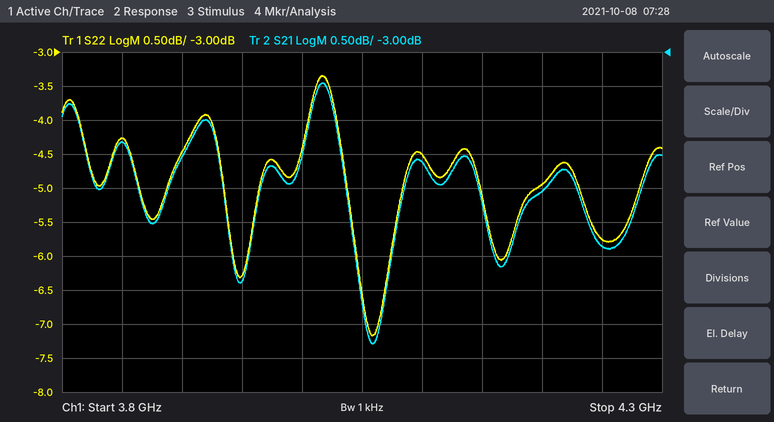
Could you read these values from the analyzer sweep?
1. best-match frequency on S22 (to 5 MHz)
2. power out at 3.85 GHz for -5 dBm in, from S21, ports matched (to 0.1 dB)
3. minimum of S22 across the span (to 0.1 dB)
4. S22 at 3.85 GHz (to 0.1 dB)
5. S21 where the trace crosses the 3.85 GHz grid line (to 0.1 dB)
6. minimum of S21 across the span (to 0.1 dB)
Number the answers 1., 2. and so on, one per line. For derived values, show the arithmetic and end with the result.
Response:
1. 4.060 GHz
2. -5 dBm + (-4.3 dB) = -9.3 dBm
3. -7.2 dB
4. -4.3 dB
5. -4.3 dB
6. -7.3 dB
